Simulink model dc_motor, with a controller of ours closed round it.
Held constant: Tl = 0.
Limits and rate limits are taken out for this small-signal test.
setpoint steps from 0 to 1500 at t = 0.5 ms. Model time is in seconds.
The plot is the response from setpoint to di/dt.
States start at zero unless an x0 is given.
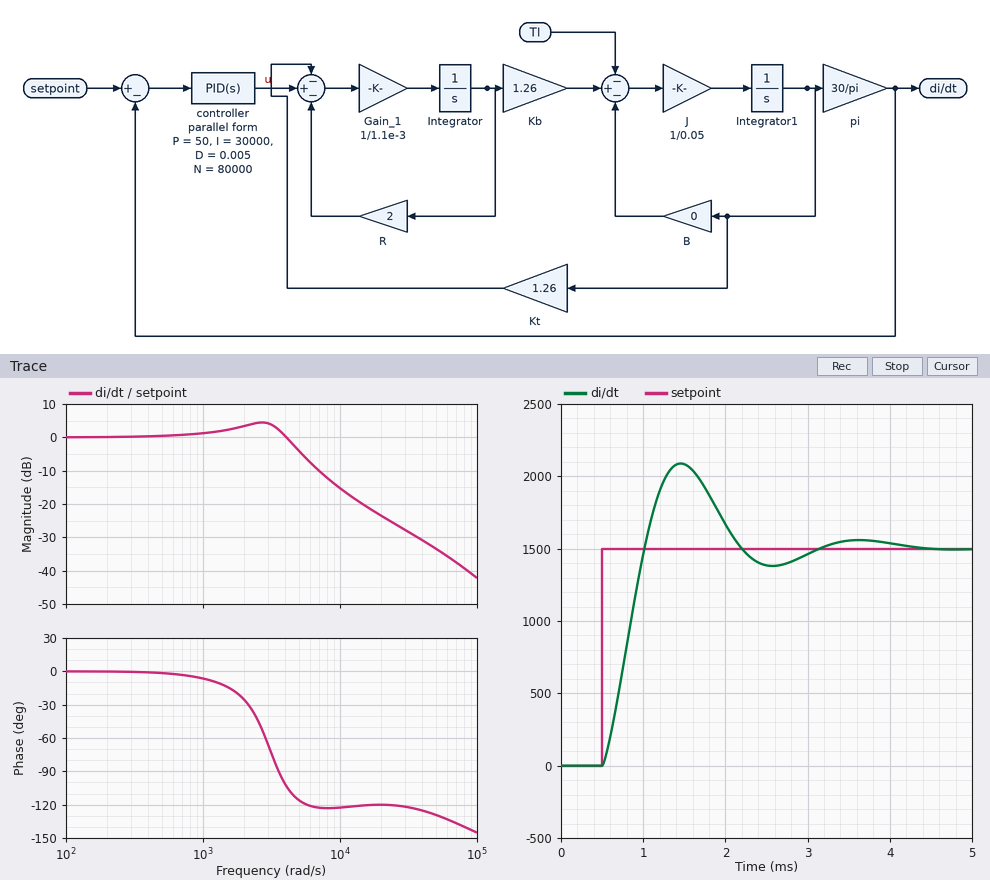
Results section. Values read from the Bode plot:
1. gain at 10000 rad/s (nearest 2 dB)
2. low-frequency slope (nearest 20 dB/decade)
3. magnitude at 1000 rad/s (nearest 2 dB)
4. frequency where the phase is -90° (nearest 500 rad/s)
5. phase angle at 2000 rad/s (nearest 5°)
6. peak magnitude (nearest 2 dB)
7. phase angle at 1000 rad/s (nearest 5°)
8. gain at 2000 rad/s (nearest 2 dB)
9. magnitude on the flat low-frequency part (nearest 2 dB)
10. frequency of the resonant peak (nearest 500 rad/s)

-16 dB
0 dB/decade
2 dB
3500 rad/s
-25°
4 dB
-5°
4 dB
0 dB
2500 rad/s
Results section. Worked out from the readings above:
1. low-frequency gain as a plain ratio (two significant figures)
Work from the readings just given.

1.0
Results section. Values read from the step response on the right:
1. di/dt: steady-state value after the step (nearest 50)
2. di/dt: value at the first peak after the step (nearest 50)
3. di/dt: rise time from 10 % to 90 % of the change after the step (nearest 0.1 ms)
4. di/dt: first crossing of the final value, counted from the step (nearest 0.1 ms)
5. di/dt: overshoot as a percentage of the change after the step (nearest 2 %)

1500
2100
0.4 ms
0.5 ms
40 %
